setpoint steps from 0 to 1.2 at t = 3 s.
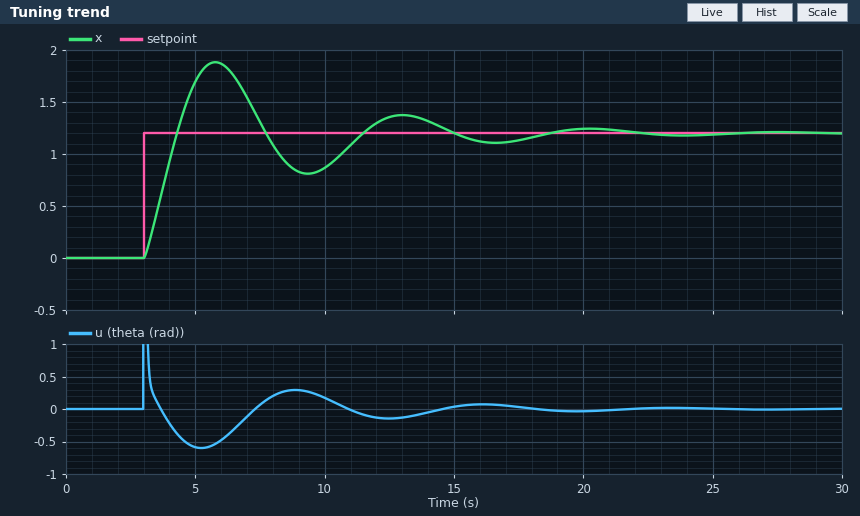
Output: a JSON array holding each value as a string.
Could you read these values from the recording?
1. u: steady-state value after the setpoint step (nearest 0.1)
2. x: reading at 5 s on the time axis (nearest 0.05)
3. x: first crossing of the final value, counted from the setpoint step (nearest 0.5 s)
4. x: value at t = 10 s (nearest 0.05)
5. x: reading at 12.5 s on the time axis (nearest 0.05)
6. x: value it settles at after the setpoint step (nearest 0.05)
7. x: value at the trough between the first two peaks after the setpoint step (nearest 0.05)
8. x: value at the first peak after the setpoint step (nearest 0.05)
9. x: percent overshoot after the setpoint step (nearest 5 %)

["0.0", "1.70", "1.5 s", "0.85", "1.35", "1.20", "0.80", "1.90", "55 %"]
